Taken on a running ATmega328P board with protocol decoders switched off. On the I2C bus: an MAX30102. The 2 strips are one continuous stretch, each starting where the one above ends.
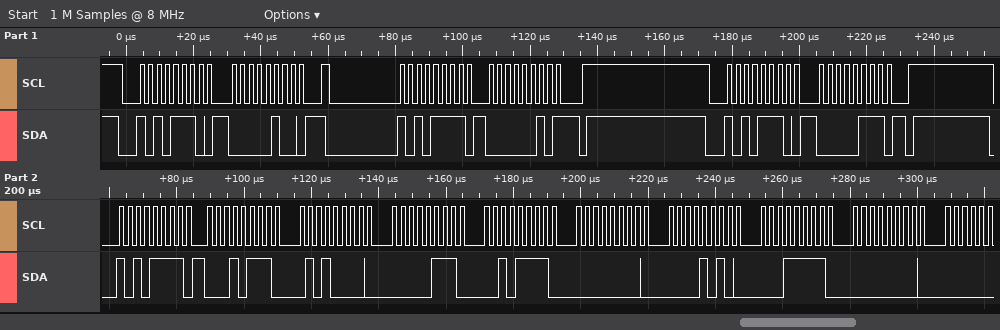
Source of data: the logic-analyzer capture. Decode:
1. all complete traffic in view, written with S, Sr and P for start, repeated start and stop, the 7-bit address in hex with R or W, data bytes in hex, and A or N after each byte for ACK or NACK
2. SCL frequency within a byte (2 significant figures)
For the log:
S 57W A 04 A Sr 57R A 02 N P S 57W A 07 A P S 57R A 17 A 50 A 07 A 2F A 00 A 0A A 1F A 00 A
400 kHz
